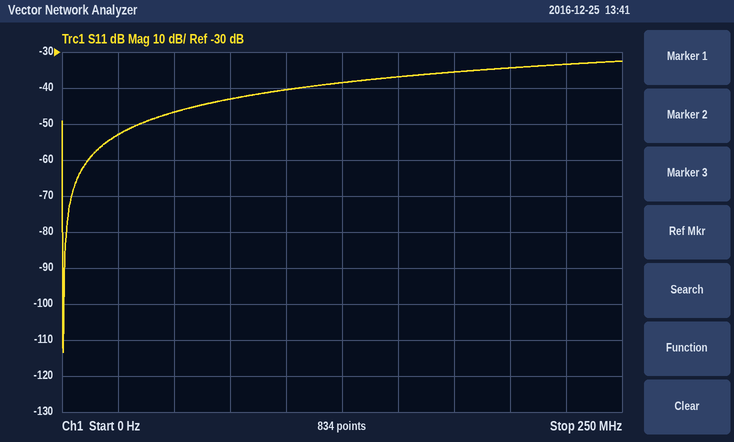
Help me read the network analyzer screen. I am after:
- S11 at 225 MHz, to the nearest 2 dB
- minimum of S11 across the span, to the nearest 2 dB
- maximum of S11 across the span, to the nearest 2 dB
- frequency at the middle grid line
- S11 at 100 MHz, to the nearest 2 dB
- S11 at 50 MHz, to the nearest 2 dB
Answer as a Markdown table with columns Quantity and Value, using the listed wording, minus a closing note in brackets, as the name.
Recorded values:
| Quantity | Value |
|---|---|
| S11 at 225 MHz, to the nearest 2 dB | -34 dB |
| minimum of S11 across the span, to the nearest 2 dB | -114 dB |
| maximum of S11 across the span, to the nearest 2 dB | -32 dB |
| frequency at the middle grid line | 125 MHz |
| S11 at 100 MHz, to the nearest 2 dB | -40 dB |
| S11 at 50 MHz, to the nearest 2 dB | -46 dB |
